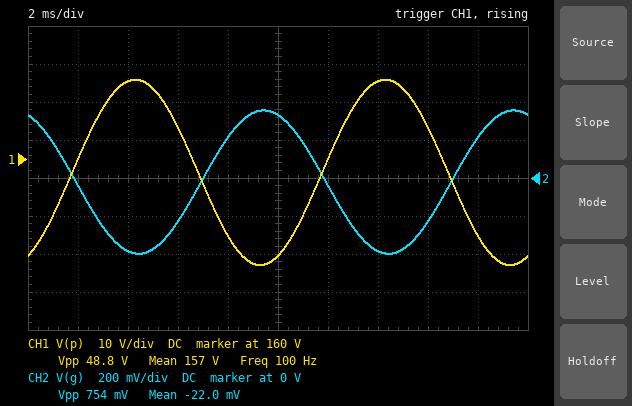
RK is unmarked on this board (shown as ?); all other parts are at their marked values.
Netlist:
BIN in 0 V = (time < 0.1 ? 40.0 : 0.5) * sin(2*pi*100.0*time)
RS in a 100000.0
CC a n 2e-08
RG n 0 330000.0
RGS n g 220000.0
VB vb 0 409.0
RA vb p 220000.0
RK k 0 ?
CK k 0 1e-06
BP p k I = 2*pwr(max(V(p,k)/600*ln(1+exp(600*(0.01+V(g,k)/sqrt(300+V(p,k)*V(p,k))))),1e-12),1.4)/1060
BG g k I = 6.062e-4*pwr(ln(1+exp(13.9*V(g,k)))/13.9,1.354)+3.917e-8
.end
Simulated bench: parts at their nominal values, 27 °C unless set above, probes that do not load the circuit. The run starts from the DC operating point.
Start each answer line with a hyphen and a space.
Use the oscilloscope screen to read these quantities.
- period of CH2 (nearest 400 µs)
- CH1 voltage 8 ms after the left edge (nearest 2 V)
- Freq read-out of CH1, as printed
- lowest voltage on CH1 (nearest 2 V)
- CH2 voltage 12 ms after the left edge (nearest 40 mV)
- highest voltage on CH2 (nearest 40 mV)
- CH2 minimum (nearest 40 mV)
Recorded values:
- 10.0 ms
- 140 V
- 100 Hz
- 132 V
- -40 mV
- 360 mV
- -400 mV
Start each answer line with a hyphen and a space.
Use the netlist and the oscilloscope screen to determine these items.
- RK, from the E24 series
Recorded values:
- 750 Ω
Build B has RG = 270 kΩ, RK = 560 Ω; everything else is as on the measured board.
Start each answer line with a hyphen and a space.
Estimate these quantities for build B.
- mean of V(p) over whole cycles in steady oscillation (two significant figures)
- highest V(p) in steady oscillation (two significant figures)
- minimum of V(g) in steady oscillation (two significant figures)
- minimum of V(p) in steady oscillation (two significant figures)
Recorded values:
- 140 V
- 170 V
- -380 mV
- 120 V
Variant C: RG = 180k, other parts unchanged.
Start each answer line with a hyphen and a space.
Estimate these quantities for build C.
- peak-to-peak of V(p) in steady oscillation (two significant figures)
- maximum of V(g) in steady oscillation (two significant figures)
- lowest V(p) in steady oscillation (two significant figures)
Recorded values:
- 40 V
- 290 mV
- 140 V
